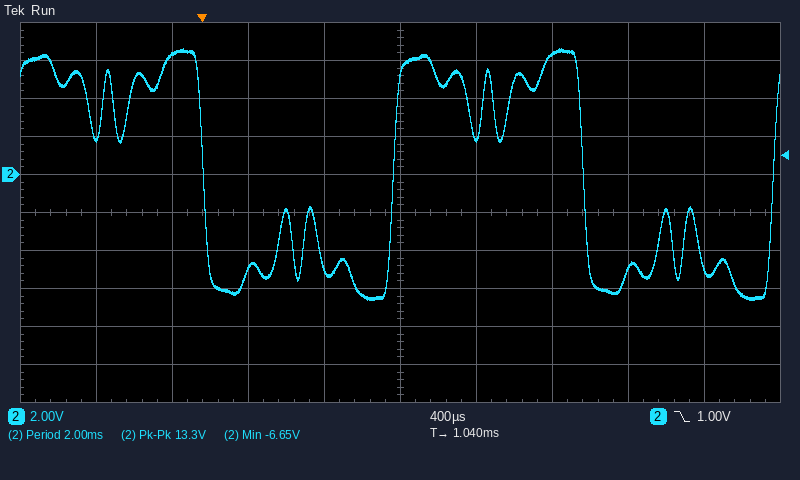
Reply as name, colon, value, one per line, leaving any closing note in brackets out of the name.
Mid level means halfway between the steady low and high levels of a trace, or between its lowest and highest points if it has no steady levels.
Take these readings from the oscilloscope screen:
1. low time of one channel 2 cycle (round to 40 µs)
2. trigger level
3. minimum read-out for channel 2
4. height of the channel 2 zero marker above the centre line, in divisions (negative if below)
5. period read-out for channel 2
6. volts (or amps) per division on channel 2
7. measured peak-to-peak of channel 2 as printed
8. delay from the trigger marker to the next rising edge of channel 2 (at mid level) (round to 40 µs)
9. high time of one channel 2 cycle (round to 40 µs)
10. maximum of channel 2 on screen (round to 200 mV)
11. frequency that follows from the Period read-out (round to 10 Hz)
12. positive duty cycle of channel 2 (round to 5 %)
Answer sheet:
low time of one channel 2 cycle: 1.00 ms
trigger level: 1.00 V
minimum read-out for channel 2: -6.65 V
height of the channel 2 zero marker above the centre line, in divisions: +1.0 div
period read-out for channel 2: 2.00 ms
volts (or amps) per division on channel 2: 2 V
measured peak-to-peak of channel 2 as printed: 13.3 V
delay from the trigger marker to the next rising edge of channel 2 (at mid level): 1.00 ms
high time of one channel 2 cycle: 1.00 ms
maximum of channel 2 on screen: 6.6 V
frequency that follows from the Period read-out: 500 Hz
positive duty cycle of channel 2: 50 %
